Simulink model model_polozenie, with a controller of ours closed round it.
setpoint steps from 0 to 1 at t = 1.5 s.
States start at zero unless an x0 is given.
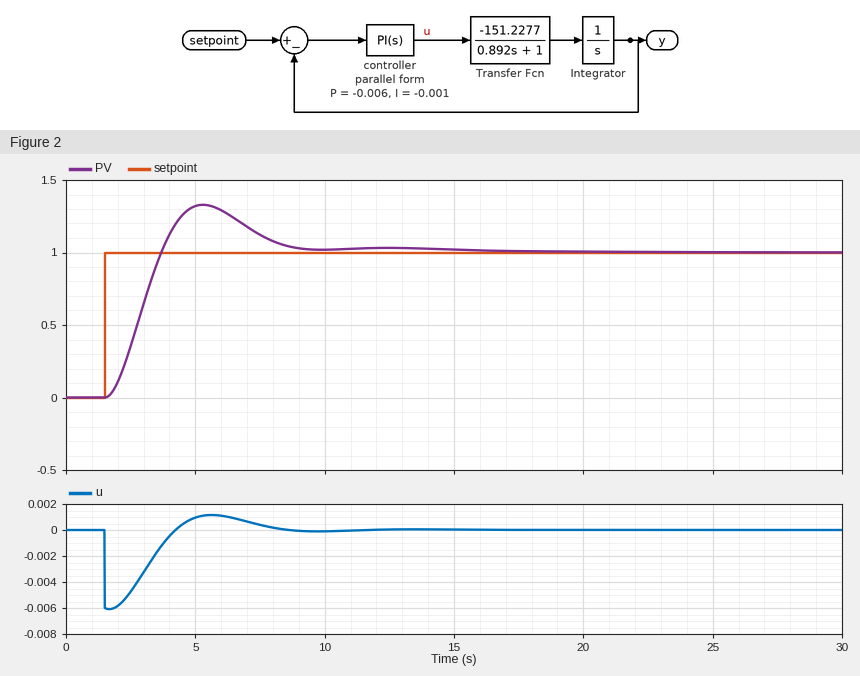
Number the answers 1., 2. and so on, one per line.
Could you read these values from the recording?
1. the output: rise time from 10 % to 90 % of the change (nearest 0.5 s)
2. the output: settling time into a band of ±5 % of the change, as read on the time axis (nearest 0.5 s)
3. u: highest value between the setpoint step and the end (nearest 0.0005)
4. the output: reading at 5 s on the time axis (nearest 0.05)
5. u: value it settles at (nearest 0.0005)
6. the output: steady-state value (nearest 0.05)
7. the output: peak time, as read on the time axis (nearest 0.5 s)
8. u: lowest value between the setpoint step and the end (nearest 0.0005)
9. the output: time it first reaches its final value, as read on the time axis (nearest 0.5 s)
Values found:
1. 1.5 s
2. 8.5 s
3. 0.0010
4. 1.30
5. 0.0000
6. 1.00
7. 5.5 s
8. -0.0060
9. 3.5 s
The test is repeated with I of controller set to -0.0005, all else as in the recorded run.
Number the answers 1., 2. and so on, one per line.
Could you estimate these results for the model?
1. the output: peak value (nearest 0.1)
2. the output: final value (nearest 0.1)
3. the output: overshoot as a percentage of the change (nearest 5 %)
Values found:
1. 1.2
2. 1.0
3. 25 %
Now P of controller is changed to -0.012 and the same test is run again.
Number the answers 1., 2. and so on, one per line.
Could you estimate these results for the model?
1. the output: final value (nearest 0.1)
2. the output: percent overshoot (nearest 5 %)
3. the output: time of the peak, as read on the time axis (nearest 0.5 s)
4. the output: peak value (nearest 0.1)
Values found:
1. 1.0
2. 35 %
3. 4.0 s
4. 1.3
